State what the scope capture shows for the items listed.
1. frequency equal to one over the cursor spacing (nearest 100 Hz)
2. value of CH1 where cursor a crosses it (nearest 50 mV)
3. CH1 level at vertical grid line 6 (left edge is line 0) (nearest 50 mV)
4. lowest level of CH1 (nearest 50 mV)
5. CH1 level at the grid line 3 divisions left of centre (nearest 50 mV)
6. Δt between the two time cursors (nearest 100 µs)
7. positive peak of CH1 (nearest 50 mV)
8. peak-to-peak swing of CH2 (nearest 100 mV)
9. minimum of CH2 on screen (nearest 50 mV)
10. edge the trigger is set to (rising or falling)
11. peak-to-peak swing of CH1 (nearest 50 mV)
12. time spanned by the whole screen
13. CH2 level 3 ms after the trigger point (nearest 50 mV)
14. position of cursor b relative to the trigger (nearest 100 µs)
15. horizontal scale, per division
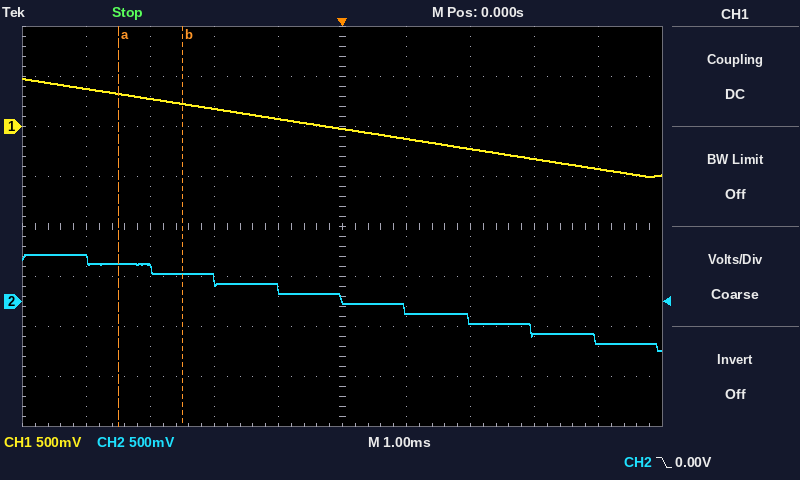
1.0 kHz
350 mV
-100 mV
-500 mV
300 mV
1.0 ms
500 mV
1.00 V
-500 mV
falling
1.00 V
10 ms
-350 mV
-2.5 ms
1 ms
